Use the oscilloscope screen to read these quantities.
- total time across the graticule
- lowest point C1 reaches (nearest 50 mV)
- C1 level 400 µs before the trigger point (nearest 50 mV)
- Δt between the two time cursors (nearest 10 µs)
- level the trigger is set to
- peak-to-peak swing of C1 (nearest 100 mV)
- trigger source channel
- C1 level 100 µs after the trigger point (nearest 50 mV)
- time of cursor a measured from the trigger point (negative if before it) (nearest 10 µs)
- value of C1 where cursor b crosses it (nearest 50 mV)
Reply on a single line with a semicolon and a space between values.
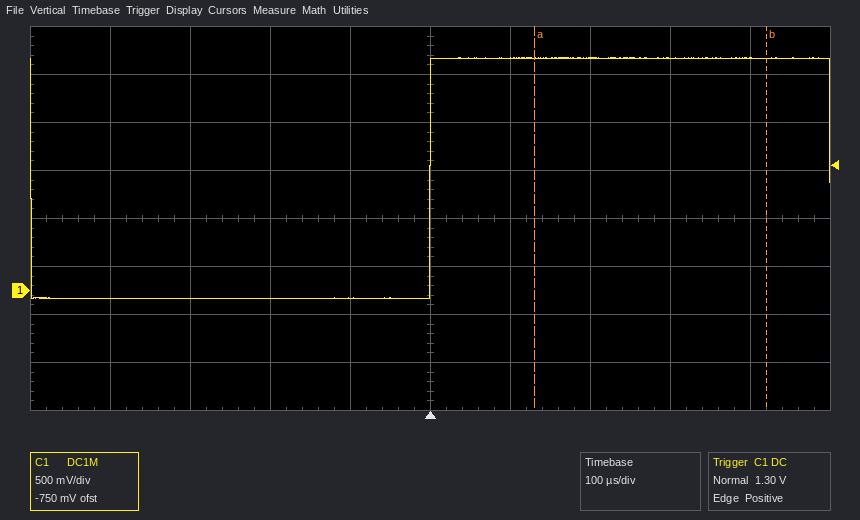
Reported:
1 ms; -100 mV; -100 mV; 290 µs; 1.30 V; 2.50 V; C1; 2.40 V; +130 µs; 2.40 V
